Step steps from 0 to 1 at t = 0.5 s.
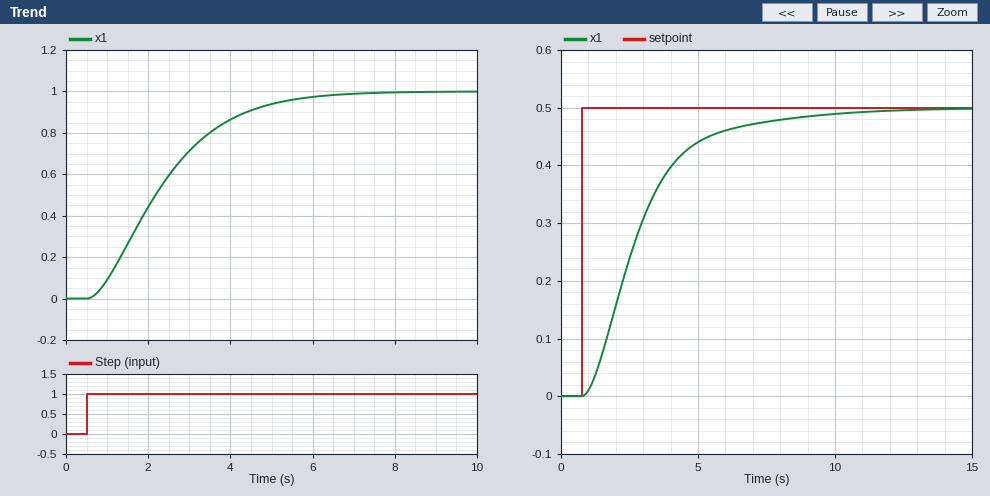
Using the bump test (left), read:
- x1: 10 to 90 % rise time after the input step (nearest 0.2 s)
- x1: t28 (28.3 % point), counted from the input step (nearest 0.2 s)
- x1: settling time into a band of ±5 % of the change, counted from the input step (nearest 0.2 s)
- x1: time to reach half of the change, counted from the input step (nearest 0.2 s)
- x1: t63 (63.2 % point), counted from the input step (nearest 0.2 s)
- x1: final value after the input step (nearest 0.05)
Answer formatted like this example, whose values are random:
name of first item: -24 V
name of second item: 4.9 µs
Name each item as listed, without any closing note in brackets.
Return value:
x1: 10 to 90 % rise time after the input step: 3.4 s
x1: t28 (28.3 % point), counted from the input step: 1.0 s
x1: settling time into a band of ±5 % of the change, counted from the input step: 4.8 s
x1: time to reach half of the change, counted from the input step: 1.6 s
x1: t63 (63.2 % point), counted from the input step: 2.2 s
x1: final value after the input step: 1.00
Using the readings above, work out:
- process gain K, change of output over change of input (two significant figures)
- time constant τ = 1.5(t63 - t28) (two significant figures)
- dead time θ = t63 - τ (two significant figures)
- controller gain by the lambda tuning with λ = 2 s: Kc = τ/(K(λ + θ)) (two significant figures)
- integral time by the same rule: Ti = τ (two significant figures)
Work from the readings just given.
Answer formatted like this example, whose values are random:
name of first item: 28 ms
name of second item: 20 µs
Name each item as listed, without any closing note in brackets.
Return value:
process gain K, change of output over change of input: 1.0
time constant τ = 1.5(t63 - t28): 1.8 s
dead time θ = t63 - τ: 0.40 s
controller gain by the lambda tuning with λ = 2 s: Kc = τ/(K(λ + θ)): 0.75
integral time by the same rule: Ti = τ: 1.8 s
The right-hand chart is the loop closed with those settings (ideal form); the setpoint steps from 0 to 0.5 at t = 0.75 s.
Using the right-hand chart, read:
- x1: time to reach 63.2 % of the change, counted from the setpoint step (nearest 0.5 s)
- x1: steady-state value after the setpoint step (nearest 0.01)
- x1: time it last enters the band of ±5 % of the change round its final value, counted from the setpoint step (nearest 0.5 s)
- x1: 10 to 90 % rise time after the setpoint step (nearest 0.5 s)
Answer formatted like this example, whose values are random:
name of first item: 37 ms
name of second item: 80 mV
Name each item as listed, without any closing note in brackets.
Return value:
x1: time to reach 63.2 % of the change, counted from the setpoint step: 2.5 s
x1: steady-state value after the setpoint step: 0.50
x1: time it last enters the band of ±5 % of the change round its final value, counted from the setpoint step: 6.5 s
x1: 10 to 90 % rise time after the setpoint step: 4.0 s
